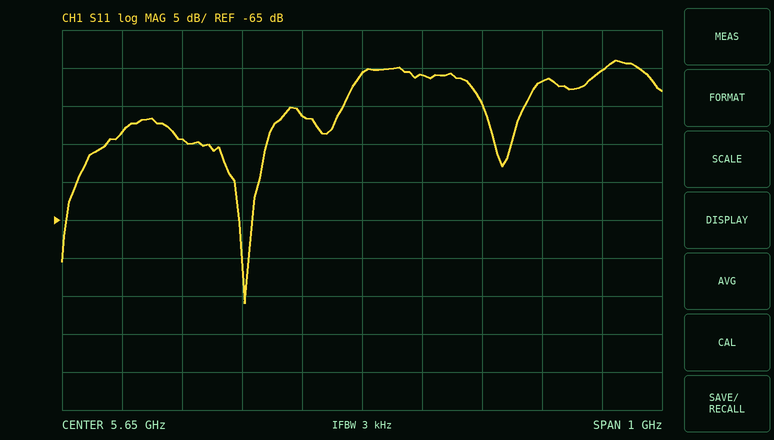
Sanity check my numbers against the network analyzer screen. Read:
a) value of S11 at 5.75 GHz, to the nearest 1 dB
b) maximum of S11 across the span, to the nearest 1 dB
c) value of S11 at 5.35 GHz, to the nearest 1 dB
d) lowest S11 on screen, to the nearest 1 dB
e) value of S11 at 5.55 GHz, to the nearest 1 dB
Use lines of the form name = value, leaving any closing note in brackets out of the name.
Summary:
value of S11 at 5.75 GHz, to the nearest 1 dB = -46 dB
maximum of S11 across the span, to the nearest 1 dB = -44 dB
value of S11 at 5.35 GHz, to the nearest 1 dB = -54 dB
lowest S11 on screen, to the nearest 1 dB = -76 dB
value of S11 at 5.55 GHz, to the nearest 1 dB = -51 dB
